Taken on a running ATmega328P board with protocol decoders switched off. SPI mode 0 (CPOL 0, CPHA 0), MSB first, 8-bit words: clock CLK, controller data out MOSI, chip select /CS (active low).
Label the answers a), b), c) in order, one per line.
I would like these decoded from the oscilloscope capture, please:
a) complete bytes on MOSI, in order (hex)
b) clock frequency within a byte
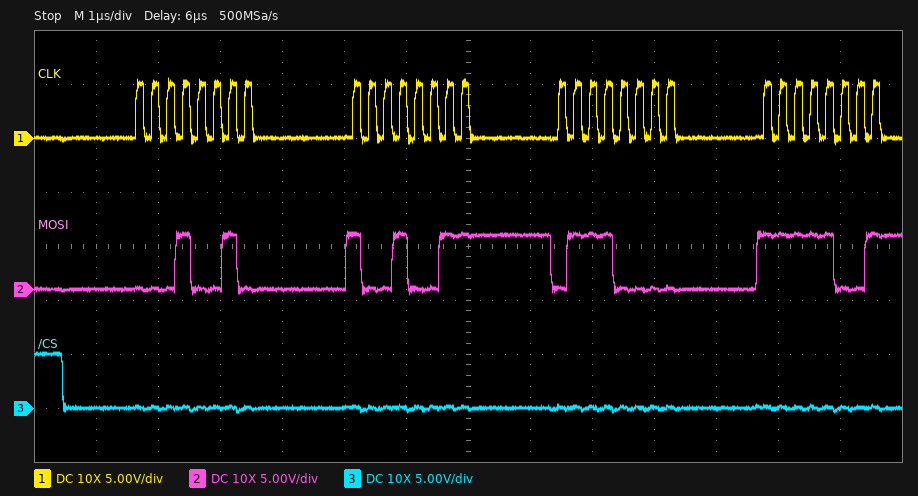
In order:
a) 0x12 0x93 0x70 0xF9
b) 4 MHz
